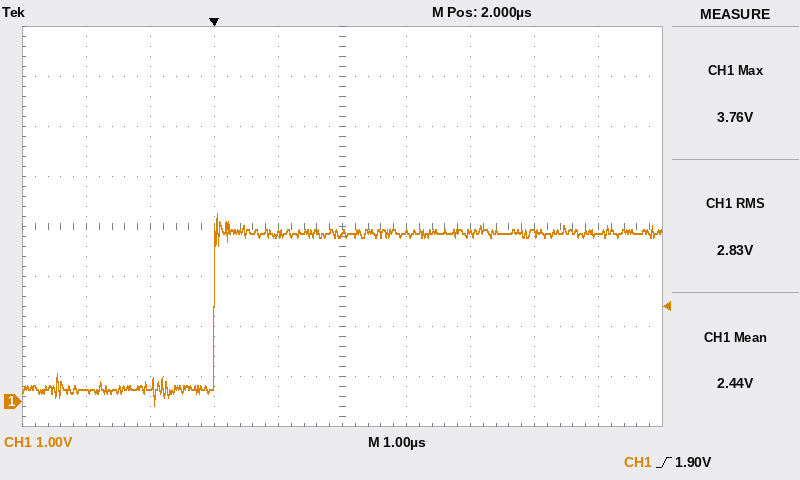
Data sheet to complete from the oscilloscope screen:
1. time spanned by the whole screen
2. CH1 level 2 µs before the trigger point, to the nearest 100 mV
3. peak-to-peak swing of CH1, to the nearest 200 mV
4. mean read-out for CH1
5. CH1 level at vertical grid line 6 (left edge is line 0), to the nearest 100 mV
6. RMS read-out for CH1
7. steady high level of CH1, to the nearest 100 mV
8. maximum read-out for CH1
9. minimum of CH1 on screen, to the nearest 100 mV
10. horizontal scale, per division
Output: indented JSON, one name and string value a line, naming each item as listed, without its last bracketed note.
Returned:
{
  "time spanned by the whole screen": "10 µs",
  "CH1 level 2 µs before the trigger point, to the nearest 100 mV": "200 mV",
  "peak-to-peak swing of CH1, to the nearest 200 mV": "3.8 V",
  "mean read-out for CH1": "2.44 V",
  "CH1 level at vertical grid line 6 (left edge is line 0), to the nearest 100 mV": "3.4 V",
  "RMS read-out for CH1": "2.83 V",
  "steady high level of CH1, to the nearest 100 mV": "3.4 V",
  "maximum read-out for CH1": "3.76 V",
  "minimum of CH1 on screen, to the nearest 100 mV": "-100 mV",
  "horizontal scale, per division": "1 µs"
}
